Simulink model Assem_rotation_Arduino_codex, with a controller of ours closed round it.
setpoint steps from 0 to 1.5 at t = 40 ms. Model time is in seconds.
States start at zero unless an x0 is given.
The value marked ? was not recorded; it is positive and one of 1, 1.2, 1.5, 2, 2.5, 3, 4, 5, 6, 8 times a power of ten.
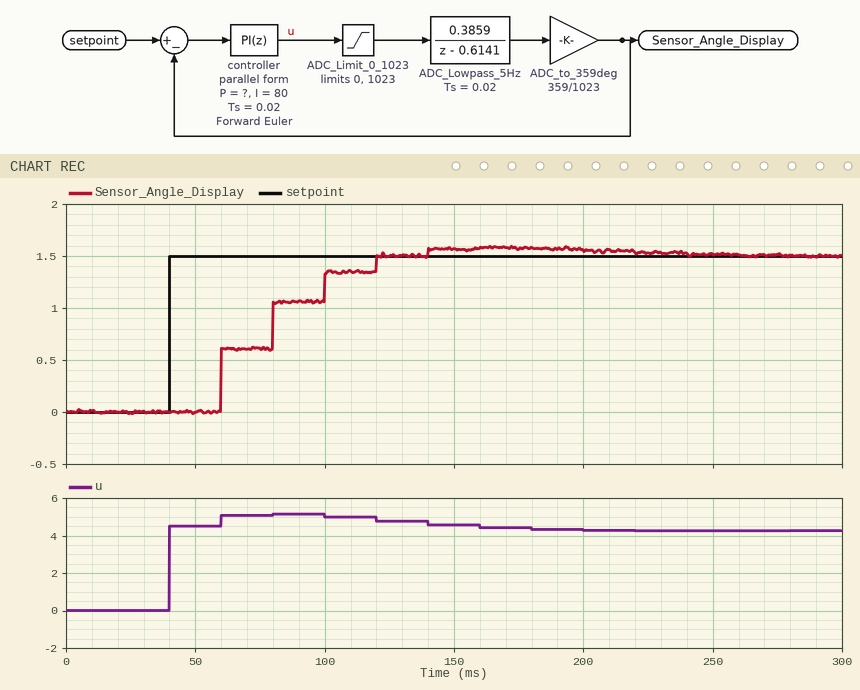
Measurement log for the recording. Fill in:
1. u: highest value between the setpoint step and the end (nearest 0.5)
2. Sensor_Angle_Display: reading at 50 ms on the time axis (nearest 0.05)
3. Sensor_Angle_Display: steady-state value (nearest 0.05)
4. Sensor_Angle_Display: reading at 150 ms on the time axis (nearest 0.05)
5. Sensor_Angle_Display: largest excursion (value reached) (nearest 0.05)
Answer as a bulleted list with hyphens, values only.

- 5.0
- 0.00
- 1.50
- 1.55
- 1.60
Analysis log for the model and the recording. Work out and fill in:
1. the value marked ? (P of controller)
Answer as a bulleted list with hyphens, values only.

- 3
